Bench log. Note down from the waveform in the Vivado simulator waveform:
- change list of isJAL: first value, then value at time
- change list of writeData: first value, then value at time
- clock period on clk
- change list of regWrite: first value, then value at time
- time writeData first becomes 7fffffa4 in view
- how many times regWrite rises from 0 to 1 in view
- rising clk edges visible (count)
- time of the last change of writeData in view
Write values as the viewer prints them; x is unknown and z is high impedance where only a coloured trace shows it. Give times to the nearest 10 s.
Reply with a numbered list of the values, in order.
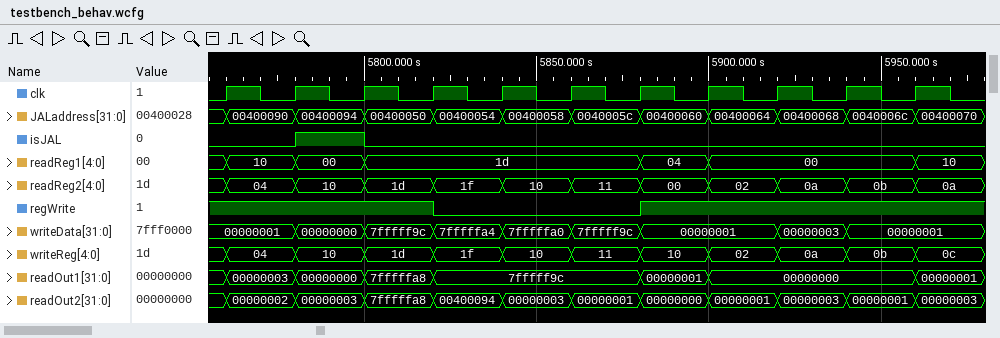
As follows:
1. 0, 1 at 5780 s, 0 at 5800 s
2. 00000001, 00000000 at 5780 s, 7fffff9c at 5800 s, 7fffffa4 at 5820 s, 7fffffa0 at 5840 s, 7fffff9c at 5860 s, 00000001 at 5880 s, 00000003 at 5920 s, 00000001 at 5940 s
3. 20 s
4. 1, 0 at 5820 s, 1 at 5880 s
5. 5820 s
6. 1
7. 11
8. 5940 s
